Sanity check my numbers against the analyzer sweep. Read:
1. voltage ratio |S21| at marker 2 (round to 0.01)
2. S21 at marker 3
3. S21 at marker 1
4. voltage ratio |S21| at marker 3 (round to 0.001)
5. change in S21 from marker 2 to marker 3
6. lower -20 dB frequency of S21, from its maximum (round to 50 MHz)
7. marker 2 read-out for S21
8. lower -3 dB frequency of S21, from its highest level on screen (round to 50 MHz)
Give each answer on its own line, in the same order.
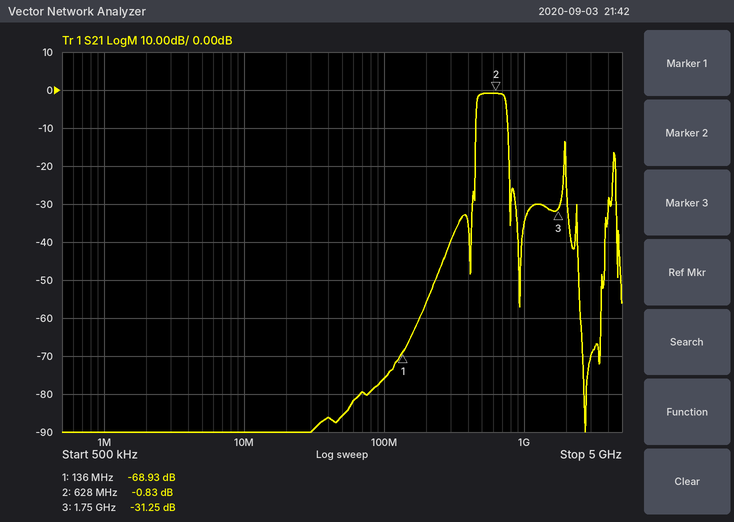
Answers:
0.91
-31.25 dB
-68.93 dB
0.027
-30.42 dB
450 MHz
-0.83 dB
450 MHz
